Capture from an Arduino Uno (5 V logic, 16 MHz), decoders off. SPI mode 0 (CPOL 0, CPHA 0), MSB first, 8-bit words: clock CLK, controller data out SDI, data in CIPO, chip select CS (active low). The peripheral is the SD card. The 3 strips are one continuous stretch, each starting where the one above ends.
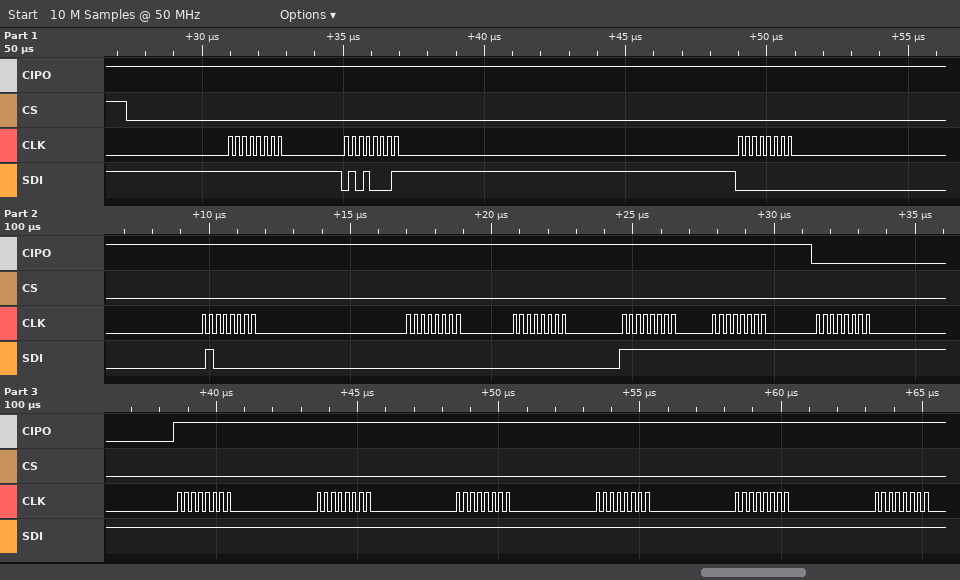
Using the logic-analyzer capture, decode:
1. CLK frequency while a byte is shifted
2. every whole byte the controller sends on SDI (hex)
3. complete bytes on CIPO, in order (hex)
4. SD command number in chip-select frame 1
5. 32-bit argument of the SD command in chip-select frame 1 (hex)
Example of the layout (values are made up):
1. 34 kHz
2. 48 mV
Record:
1. 4 MHz
2. 0xFF 0x51 0x00 0x40 0x00 0x00 0xFF 0xFF 0xFF 0xFF 0xFF 0xFF 0xFF 0xFF 0xFF
3. 0xFF 0xFF 0xFF 0xFF 0xFF 0xFF 0xFF 0xFF 0x00 0xFF 0xFF 0xFF 0xFF 0xFF 0xFF
4. CMD17
5. 0x00400000
